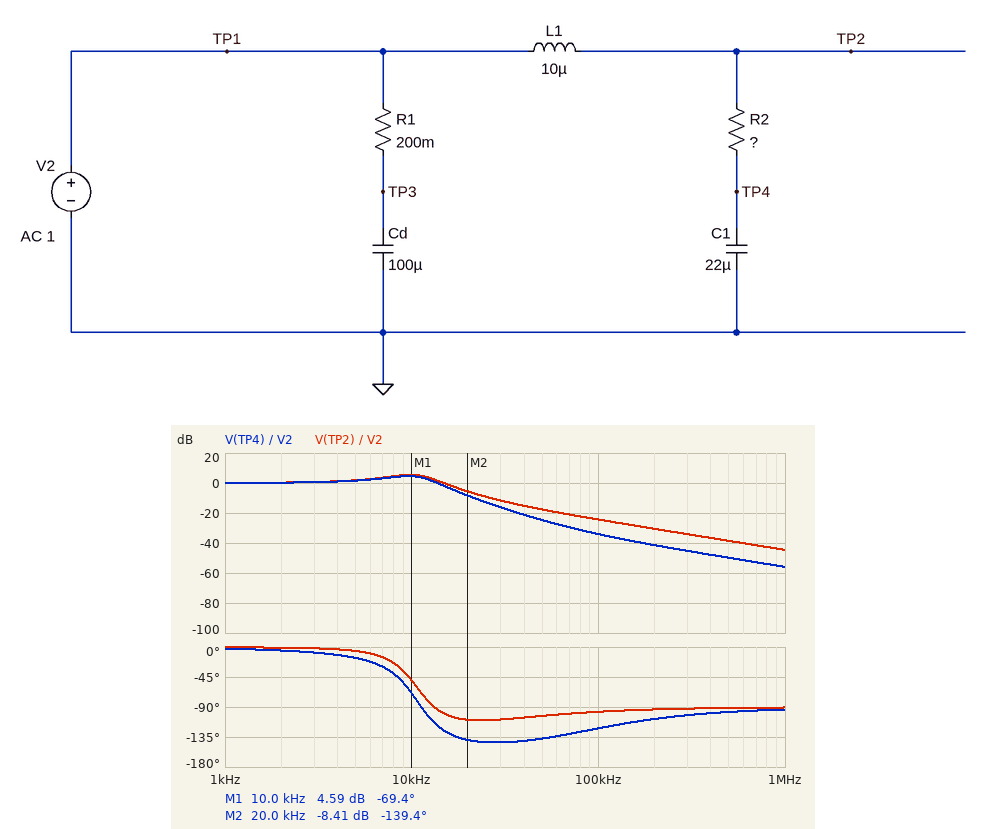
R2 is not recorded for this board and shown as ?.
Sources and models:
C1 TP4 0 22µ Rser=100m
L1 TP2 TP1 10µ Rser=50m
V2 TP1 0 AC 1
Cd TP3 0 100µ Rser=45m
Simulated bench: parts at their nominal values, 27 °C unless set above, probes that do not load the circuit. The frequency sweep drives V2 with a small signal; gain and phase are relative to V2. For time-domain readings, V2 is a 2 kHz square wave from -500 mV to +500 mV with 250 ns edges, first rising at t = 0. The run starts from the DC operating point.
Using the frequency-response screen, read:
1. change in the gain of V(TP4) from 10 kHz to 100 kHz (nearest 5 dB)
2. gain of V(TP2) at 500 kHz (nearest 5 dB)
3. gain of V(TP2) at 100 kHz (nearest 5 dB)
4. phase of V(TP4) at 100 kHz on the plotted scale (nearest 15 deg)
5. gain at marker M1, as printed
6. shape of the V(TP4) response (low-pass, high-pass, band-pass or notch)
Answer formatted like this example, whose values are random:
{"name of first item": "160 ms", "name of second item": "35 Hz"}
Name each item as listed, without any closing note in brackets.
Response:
{"change in the gain of V(TP4) from 10 kHz to 100 kHz": "-40 dB", "gain of V(TP2) at 500 kHz": "-40 dB", "gain of V(TP2) at 100 kHz": "-25 dB", "phase of V(TP4) at 100 kHz on the plotted scale": "-120 deg", "gain at marker M1, as printed": "4.59 dB", "shape of the V(TP4) response": "low-pass"}
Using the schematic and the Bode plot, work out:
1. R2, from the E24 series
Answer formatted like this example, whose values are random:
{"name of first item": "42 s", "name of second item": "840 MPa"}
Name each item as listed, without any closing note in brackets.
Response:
{"R2, from the E24 series": "0.27 Ω"}
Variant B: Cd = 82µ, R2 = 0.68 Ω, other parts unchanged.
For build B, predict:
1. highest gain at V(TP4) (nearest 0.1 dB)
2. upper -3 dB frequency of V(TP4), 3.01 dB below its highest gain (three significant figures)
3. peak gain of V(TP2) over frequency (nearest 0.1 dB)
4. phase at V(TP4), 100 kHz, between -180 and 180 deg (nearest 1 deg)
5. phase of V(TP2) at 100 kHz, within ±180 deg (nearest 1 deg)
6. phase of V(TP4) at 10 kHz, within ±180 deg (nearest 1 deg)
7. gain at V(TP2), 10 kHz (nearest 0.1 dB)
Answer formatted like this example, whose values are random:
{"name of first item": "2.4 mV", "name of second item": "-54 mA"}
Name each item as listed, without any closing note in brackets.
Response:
{"highest gain at V(TP4)": "0.3 dB", "upper -3 dB frequency of V(TP4), 3.01 dB below its highest gain": "11.9 kHz", "peak gain of V(TP2) over frequency": "2.3 dB", "phase at V(TP4), 100 kHz, between -180 and 180 deg": "-118 deg", "phase of V(TP2) at 100 kHz, within ±180 deg": "-88 deg", "phase of V(TP4) at 10 kHz, within ±180 deg": "-76 deg", "gain at V(TP2), 10 kHz": "2.1 dB"}
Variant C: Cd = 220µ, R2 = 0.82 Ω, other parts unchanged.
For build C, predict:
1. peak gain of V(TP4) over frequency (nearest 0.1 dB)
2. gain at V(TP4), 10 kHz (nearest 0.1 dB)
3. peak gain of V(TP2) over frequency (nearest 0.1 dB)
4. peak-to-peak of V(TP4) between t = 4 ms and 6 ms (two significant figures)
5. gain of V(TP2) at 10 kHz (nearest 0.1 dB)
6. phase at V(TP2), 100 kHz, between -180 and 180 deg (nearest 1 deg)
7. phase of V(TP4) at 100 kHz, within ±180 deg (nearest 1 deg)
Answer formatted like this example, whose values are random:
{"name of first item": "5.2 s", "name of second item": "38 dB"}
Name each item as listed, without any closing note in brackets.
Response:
{"peak gain of V(TP4) over frequency": "0 dB", "gain at V(TP4), 10 kHz": "-2.5 dB", "peak gain of V(TP2) over frequency": "1.8 dB", "peak-to-peak of V(TP4) between t = 4 ms and 6 ms": "1.1 V", "gain of V(TP2) at 10 kHz": "1.6 dB", "phase at V(TP2), 100 kHz, between -180 and 180 deg": "-86 deg", "phase of V(TP4) at 100 kHz, within ±180 deg": "-117 deg"}
